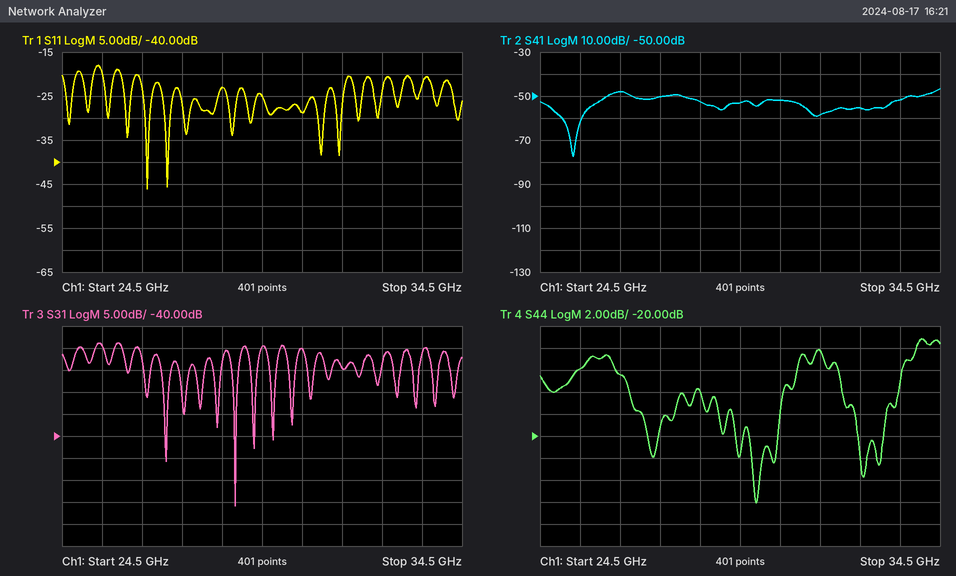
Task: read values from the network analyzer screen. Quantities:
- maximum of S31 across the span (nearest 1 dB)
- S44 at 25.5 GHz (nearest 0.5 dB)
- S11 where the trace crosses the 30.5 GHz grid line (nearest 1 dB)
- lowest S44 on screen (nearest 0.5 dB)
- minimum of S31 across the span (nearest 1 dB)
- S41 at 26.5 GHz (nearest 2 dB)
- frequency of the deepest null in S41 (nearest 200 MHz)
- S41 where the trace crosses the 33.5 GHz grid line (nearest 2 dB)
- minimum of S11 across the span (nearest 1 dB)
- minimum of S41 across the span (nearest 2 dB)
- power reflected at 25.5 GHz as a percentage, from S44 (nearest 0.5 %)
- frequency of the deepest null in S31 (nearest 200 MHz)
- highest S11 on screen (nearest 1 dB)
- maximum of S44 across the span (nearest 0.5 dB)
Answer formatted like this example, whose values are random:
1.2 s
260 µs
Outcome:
-19 dB
-14.0 dB
-29 dB
-26.0 dB
-56 dB
-48 dB
25.4 GHz
-52 dB
-46 dB
-78 dB
4.0 %
28.8 GHz
-18 dB
-11.0 dB
